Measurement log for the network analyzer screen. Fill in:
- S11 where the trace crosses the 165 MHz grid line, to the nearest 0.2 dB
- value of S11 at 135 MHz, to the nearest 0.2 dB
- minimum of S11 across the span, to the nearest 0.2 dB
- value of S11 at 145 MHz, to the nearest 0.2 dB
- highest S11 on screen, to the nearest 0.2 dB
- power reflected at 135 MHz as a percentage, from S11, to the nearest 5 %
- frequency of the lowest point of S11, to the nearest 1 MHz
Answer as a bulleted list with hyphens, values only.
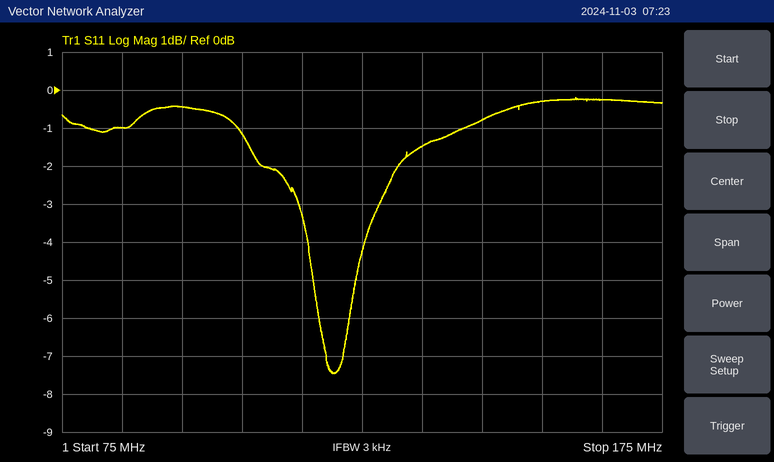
- -0.2 dB
- -1.4 dB
- -7.4 dB
- -0.8 dB
- -0.2 dB
- 70 %
- 120 MHz
